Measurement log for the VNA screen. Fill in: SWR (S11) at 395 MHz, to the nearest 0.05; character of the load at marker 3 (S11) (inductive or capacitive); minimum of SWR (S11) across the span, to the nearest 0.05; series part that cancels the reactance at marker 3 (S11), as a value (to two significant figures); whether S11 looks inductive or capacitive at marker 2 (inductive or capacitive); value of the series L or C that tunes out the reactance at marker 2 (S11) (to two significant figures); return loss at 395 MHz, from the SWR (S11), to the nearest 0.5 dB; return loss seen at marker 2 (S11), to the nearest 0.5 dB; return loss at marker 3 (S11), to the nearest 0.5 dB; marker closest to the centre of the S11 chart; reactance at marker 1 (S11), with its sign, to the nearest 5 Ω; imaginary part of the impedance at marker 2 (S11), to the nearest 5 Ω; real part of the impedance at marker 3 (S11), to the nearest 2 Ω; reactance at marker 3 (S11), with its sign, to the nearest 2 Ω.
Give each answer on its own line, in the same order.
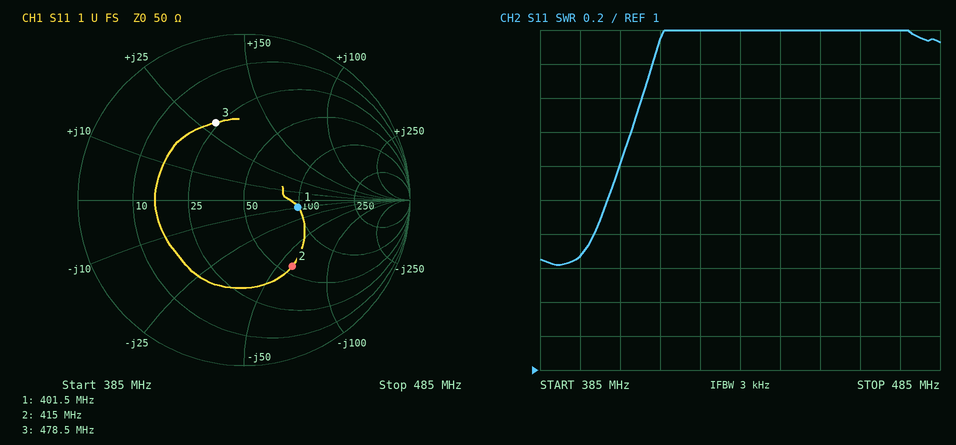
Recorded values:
1.65
inductive
1.60
11 pF
capacitive
23 nH
12.0 dB
6.0 dB
6.0 dB
marker 1
-10 Ω
-60 Ω
24 Ω
+30 Ω
